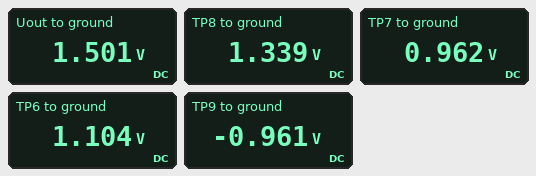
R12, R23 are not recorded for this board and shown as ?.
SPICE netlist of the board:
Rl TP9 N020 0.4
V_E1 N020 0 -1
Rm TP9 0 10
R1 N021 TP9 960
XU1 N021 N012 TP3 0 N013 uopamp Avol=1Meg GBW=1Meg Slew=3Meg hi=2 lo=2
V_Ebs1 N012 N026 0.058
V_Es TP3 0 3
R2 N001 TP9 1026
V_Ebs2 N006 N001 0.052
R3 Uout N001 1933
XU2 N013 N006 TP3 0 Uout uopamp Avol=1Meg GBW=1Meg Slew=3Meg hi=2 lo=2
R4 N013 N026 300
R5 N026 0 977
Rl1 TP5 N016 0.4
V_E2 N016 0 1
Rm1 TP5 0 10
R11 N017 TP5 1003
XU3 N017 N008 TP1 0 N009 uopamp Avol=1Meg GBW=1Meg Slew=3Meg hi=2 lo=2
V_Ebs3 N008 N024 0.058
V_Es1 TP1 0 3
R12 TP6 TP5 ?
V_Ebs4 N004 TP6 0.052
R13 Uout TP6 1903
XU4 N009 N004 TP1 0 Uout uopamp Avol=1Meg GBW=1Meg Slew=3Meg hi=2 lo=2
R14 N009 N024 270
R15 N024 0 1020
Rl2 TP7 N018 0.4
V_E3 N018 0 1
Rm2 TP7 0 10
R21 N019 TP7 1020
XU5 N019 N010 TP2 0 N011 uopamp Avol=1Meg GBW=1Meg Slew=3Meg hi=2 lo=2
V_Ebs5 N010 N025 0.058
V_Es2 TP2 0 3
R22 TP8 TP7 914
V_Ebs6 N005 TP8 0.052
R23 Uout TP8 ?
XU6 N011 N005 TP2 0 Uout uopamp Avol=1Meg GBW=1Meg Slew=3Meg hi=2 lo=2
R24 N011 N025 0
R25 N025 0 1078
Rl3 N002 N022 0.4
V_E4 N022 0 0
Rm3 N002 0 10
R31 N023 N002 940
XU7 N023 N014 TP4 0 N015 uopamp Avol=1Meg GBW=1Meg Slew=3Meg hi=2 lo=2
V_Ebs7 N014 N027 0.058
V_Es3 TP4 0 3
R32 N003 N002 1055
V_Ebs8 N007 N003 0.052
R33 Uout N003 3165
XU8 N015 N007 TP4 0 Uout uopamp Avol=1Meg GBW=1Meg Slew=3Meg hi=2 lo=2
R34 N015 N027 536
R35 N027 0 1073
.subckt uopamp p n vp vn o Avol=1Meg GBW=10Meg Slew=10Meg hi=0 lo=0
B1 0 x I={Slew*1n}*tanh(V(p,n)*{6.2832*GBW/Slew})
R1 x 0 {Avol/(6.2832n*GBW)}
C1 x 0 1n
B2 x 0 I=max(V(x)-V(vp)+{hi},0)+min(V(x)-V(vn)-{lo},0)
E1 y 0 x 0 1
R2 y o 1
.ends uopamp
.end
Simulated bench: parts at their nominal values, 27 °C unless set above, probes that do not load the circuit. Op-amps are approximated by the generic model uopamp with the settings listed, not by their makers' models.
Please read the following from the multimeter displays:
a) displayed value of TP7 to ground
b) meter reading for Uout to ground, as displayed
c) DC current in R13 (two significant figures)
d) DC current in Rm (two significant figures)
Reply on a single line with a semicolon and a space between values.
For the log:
0.962 V; 1.501 V; 210 µA; 96 mA
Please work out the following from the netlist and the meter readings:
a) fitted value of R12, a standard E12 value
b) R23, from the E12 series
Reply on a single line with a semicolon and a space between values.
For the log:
680 Ω; 390 Ω
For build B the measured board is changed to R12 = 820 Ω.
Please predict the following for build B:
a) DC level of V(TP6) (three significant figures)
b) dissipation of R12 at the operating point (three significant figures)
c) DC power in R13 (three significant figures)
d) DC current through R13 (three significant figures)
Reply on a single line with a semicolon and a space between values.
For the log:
1.12 V; 32.1 µW; 74.6 µW; 198 µA
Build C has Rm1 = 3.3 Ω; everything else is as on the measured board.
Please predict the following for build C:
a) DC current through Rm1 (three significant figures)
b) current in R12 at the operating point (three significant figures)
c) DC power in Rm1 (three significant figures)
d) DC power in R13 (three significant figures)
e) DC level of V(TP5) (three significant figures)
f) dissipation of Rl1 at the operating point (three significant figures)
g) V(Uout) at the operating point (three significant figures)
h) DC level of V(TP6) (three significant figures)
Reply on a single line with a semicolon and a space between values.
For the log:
270 mA; 236 µA; 241 mW; 106 µW; 892 mV; 29.2 mW; 1.50 V; 1.05 V
